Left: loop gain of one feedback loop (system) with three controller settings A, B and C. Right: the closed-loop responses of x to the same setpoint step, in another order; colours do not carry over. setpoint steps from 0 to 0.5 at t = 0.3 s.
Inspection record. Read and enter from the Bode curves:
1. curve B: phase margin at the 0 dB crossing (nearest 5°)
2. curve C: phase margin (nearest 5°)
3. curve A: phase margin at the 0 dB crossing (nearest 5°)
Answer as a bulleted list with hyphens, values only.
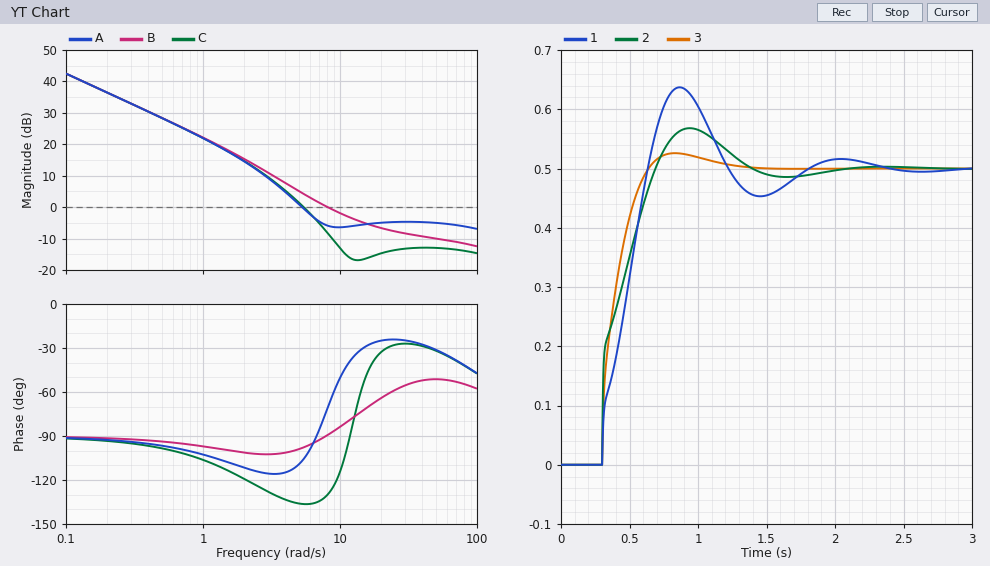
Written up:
- 90°
- 45°
- 75°
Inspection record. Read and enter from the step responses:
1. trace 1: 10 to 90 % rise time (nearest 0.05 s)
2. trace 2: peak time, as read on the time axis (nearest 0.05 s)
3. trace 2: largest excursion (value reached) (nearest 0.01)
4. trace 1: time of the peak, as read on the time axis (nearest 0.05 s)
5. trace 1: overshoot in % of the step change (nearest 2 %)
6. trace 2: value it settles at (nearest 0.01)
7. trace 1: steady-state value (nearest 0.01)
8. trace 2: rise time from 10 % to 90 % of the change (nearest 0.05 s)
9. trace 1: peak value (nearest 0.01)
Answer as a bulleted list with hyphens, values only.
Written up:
- 0.30 s
- 0.95 s
- 0.57
- 0.85 s
- 28 %
- 0.50
- 0.50
- 0.30 s
- 0.64
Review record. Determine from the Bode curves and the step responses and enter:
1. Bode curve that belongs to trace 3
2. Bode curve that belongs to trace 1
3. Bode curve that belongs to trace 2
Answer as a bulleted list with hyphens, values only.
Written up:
- B
- C
- A
